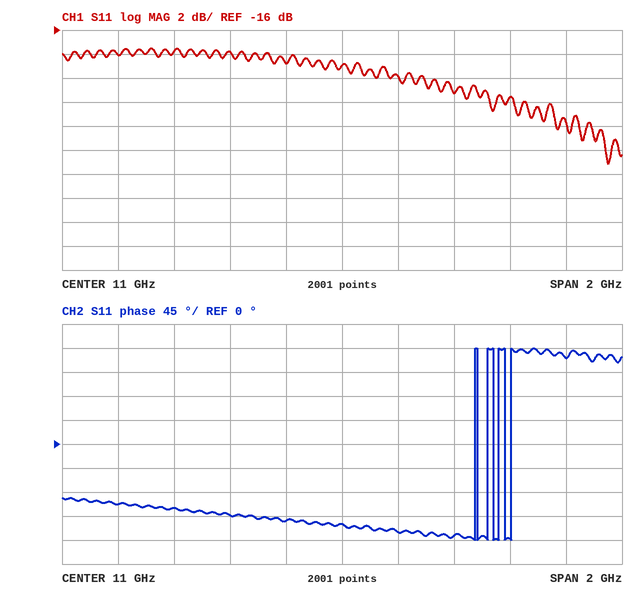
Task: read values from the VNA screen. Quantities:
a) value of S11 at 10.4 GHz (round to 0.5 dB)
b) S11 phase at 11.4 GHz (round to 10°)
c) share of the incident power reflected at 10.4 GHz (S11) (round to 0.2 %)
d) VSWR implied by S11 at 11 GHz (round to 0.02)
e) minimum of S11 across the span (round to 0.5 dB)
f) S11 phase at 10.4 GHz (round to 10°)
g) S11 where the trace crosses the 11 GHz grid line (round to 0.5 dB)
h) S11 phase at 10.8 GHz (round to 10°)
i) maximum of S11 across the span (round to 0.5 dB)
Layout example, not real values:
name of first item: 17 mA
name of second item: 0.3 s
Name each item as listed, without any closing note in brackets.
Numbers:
value of S11 at 10.4 GHz: -18.0 dB
S11 phase at 11.4 GHz: -170°
share of the incident power reflected at 10.4 GHz (S11): 1.6 %
VSWR implied by S11 at 11 GHz: 1.26
minimum of S11 across the span: -27.0 dB
S11 phase at 10.4 GHz: -120°
S11 where the trace crosses the 11 GHz grid line: -19.0 dB
S11 phase at 10.8 GHz: -140°
maximum of S11 across the span: -17.5 dB
